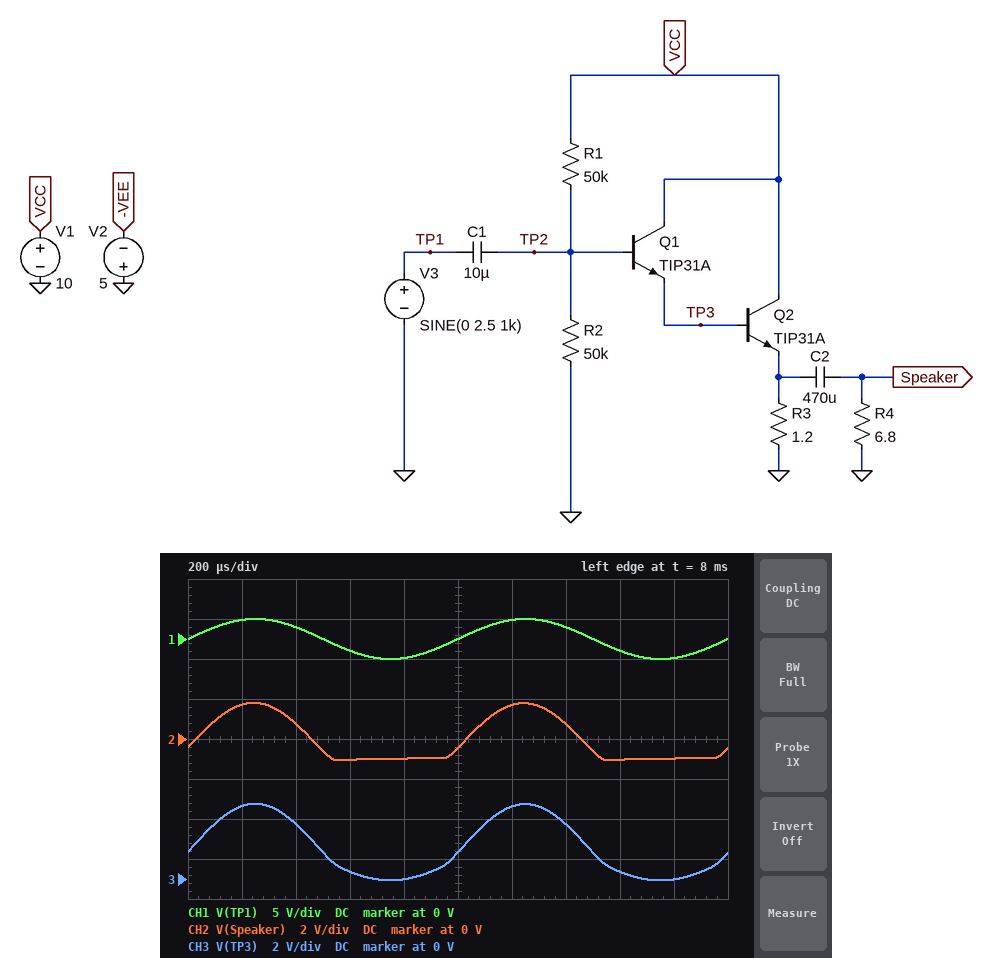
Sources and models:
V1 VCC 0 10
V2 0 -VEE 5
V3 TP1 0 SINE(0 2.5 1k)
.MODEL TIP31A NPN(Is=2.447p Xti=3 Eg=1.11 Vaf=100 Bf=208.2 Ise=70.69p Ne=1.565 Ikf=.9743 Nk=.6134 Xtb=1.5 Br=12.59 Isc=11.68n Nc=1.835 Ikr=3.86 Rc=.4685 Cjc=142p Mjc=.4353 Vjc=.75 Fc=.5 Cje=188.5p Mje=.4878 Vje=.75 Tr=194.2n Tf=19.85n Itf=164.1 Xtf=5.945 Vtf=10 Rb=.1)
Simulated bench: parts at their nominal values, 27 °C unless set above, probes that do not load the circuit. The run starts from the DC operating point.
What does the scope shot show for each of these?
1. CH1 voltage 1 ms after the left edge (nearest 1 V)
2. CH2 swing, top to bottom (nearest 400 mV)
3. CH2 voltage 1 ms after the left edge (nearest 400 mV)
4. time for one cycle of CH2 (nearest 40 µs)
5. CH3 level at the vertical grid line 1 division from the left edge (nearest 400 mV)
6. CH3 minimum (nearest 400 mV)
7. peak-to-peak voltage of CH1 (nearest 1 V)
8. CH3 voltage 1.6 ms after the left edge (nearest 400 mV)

0 V
2.8 V
-400 mV
1.00 ms
3.6 V
0 V
5 V
400 mV
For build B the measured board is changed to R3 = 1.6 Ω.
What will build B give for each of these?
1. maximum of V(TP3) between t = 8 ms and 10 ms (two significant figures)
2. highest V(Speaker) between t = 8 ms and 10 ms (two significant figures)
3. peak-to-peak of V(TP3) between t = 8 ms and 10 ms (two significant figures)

4.0 V
1.9 V
3.9 V
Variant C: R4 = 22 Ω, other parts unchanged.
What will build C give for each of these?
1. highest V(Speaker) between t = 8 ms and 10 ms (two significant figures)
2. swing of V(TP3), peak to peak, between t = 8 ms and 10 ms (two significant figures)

2.0 V
3.9 V
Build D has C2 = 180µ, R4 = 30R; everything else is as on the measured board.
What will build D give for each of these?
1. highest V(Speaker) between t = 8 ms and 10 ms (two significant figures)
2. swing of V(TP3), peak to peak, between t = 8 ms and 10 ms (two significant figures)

1.9 V
3.9 V
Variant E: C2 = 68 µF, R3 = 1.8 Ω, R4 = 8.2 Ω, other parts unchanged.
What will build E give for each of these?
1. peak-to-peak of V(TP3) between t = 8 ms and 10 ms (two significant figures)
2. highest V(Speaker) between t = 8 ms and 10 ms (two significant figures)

4.0 V
1.9 V
